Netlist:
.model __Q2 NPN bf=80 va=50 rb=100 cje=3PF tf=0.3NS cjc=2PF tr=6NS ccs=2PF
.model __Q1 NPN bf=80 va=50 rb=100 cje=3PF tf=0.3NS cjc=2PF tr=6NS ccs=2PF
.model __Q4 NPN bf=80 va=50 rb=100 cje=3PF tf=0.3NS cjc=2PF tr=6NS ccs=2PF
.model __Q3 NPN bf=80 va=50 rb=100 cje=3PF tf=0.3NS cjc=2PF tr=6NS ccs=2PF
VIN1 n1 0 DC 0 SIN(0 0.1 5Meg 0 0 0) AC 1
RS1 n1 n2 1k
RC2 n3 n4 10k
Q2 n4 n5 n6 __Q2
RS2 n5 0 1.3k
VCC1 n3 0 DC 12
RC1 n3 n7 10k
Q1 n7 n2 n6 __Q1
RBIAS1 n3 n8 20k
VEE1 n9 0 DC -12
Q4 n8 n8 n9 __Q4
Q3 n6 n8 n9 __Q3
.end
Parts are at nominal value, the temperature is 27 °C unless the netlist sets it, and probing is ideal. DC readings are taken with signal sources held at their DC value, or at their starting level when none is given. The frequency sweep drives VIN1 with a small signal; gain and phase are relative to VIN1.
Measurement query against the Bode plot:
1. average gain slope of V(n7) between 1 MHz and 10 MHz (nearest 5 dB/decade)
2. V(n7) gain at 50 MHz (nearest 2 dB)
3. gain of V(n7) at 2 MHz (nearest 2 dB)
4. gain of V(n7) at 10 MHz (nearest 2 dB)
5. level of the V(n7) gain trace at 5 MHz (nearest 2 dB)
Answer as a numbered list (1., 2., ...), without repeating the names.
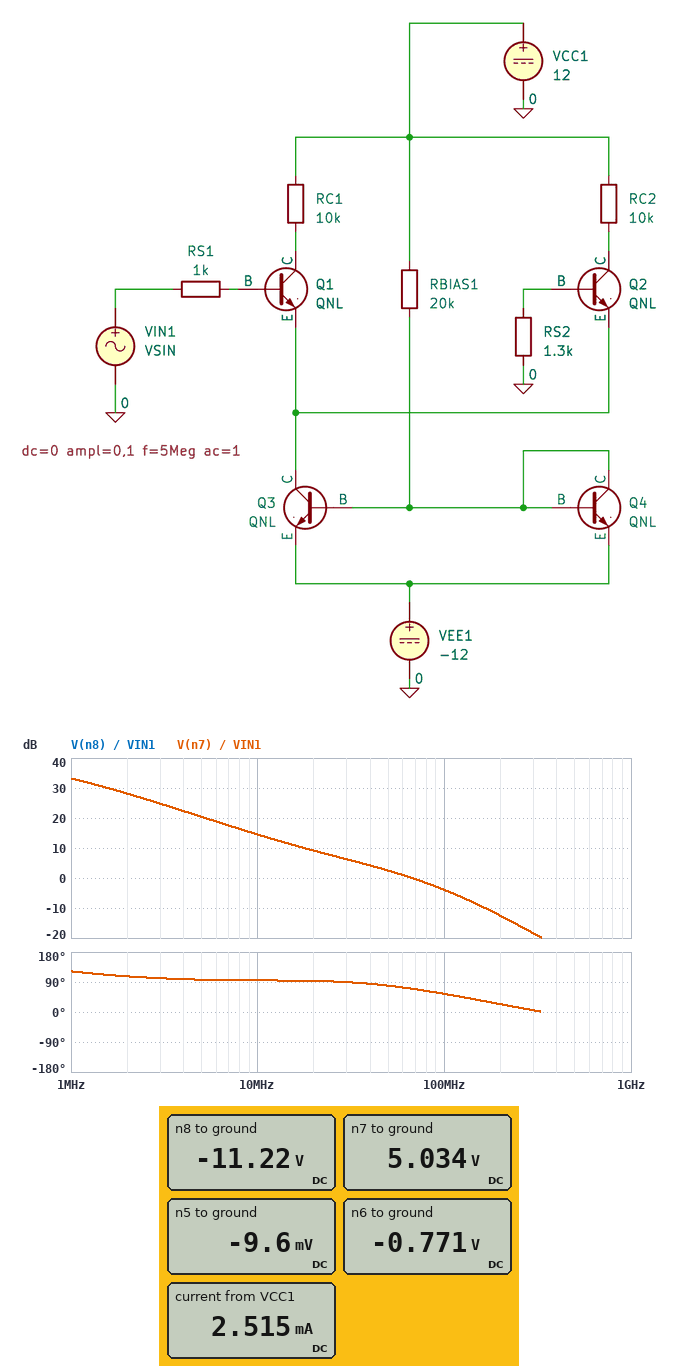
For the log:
1. -20 dB/decade
2. 2 dB
3. 28 dB
4. 14 dB
5. 20 dB
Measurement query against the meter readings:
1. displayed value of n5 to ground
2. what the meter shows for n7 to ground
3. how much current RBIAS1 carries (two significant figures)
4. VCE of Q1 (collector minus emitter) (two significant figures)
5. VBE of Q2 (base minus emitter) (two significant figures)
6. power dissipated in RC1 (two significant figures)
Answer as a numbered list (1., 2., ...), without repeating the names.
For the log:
1. -9.6 mV
2. 5.034 V
3. 1.2 mA
4. 5.8 V
5. 760 mV
6. 4.9 mW
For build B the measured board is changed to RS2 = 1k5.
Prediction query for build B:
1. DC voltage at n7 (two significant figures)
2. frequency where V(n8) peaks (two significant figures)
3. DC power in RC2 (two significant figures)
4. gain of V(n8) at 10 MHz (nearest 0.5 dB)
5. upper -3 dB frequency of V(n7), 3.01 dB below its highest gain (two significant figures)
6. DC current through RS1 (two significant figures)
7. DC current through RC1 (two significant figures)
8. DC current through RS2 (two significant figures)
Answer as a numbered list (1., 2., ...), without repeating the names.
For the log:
1. 4.9 V
2. 120 MHz
3. 4.2 mW
4. -63.5 dB
5. 600 kHz
6. 8.1 µA
7. 710 µA
8. 7.3 µA
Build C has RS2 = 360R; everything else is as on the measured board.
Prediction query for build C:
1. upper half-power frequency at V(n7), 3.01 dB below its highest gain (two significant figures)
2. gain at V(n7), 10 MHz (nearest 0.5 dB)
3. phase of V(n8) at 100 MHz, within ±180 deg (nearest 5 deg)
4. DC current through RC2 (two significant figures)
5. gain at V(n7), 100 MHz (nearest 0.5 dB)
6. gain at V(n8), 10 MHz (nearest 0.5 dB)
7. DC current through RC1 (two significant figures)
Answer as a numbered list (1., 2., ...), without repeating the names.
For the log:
1. 880 kHz
2. 18.5 dB
3. 10 deg
4. 720 µA
5. -3.0 dB
6. -68.5 dB
7. 630 µA
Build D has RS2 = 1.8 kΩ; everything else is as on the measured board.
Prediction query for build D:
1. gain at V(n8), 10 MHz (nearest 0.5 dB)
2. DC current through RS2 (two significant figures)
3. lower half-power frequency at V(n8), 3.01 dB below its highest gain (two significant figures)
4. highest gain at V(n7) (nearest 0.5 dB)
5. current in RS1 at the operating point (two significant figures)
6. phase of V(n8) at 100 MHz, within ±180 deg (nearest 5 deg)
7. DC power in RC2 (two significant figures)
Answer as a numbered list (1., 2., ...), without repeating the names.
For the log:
1. -63.0 dB
2. 7.0 µA
3. 39 MHz
4. 38.0 dB
5. 8.3 µA
6. -5 deg
7. 3.9 mW
